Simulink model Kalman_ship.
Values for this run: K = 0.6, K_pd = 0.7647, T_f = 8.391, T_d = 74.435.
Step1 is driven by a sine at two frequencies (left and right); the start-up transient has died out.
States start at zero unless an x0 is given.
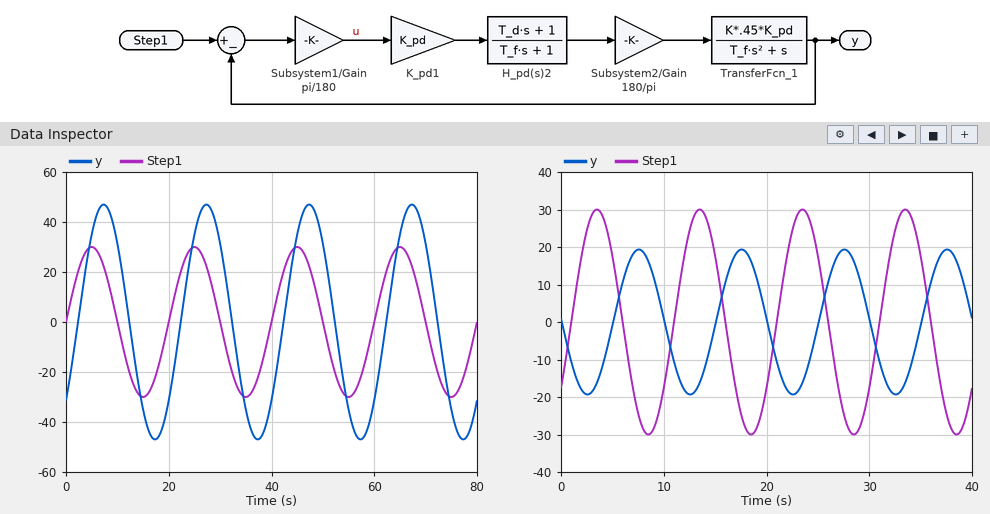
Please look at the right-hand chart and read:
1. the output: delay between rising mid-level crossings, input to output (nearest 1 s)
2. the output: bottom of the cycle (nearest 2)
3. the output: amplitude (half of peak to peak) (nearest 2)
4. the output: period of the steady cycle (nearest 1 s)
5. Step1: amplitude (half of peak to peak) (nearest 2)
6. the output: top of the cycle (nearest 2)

4 s
-20
20
10 s
30
20
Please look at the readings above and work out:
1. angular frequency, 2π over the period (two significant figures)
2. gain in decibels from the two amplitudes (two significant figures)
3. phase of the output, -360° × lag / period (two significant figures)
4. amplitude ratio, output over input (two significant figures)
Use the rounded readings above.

0.63 rad/s
-3.5 dB
-140°
0.67
